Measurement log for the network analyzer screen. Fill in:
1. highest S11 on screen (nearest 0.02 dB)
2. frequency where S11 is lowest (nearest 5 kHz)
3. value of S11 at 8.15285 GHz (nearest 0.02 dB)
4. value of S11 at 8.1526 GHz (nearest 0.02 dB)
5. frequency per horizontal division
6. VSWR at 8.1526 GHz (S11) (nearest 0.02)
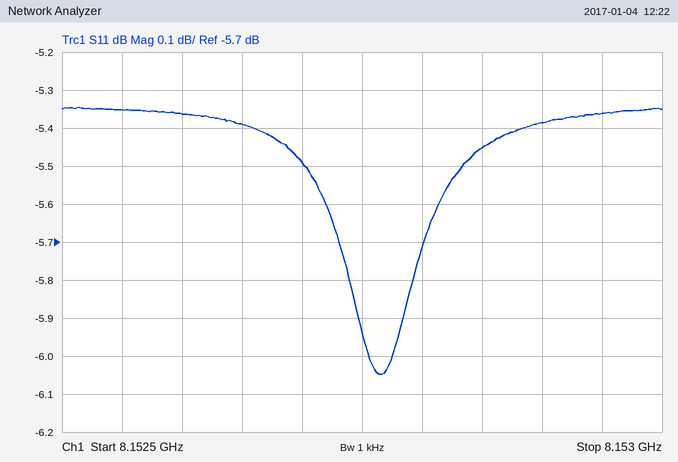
-5.34 dB
8.152765 GHz
-5.46 dB
-5.36 dB
50 kHz
3.34
